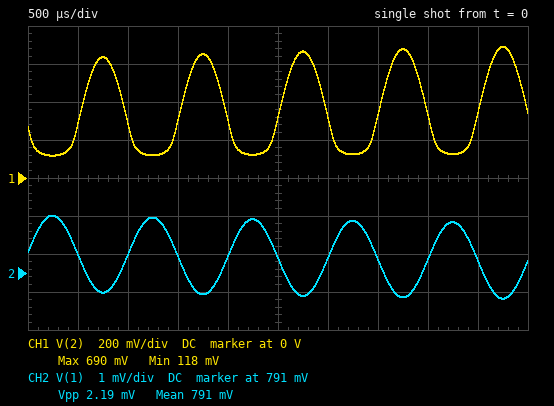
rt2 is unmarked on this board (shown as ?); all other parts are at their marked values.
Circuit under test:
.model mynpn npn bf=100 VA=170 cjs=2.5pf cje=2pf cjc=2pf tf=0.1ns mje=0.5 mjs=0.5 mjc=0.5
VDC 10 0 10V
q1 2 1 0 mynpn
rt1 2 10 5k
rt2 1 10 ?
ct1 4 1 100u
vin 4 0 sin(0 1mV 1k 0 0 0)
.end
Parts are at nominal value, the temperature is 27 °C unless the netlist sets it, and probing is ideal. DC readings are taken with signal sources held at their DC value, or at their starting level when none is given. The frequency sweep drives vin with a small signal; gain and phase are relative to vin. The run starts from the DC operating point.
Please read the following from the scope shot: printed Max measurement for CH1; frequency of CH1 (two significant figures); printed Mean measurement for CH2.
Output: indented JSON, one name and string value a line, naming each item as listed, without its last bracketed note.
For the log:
{
  "printed Max measurement for CH1": "690 mV",
  "frequency of CH1": "1.0 kHz",
  "printed Mean measurement for CH2": "791 mV"
}
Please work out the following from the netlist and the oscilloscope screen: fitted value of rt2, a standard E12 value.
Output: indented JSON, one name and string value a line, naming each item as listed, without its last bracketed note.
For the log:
{
  "fitted value of rt2, a standard E12 value": "470 kΩ"
}
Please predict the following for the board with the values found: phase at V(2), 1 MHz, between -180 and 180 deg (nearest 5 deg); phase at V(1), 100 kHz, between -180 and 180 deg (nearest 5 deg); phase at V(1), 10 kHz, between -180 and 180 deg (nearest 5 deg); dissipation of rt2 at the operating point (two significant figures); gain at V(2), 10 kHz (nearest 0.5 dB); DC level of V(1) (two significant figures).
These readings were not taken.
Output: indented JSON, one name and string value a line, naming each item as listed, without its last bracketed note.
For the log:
{
  "phase at V(2), 1 MHz, between -180 and 180 deg": "170 deg",
  "phase at V(1), 100 kHz, between -180 and 180 deg": "0 deg",
  "phase at V(1), 10 kHz, between -180 and 180 deg": "0 deg",
  "dissipation of rt2 at the operating point": "180 µW",
  "gain at V(2), 10 kHz": "51.0 dB",
  "DC level of V(1)": "790 mV"
}
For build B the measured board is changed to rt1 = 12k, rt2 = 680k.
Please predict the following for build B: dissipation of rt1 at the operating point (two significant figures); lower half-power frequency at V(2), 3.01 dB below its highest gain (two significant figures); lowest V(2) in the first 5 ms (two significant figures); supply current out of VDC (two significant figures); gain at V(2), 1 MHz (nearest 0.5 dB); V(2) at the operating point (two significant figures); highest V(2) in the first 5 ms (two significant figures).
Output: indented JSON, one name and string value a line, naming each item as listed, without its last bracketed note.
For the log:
{
  "dissipation of rt1 at the operating point": "8.1 mW",
  "lower half-power frequency at V(2), 3.01 dB below its highest gain": "22 Hz",
  "lowest V(2) in the first 5 ms": "98 mV",
  "supply current out of VDC": "840 µA",
  "gain at V(2), 1 MHz": "36.0 dB",
  "V(2) at the operating point": "130 mV",
  "highest V(2) in the first 5 ms": "410 mV"
}
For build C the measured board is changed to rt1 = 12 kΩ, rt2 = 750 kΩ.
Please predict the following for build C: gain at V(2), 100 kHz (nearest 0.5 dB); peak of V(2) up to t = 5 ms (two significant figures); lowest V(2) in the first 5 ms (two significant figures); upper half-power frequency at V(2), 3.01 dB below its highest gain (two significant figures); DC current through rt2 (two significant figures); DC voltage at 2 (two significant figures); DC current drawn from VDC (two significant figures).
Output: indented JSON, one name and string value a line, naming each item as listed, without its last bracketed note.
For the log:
{
  "gain at V(2), 100 kHz": "38.0 dB",
  "peak of V(2) up to t = 5 ms": "450 mV",
  "lowest V(2) in the first 5 ms": "100 mV",
  "upper half-power frequency at V(2), 3.01 dB below its highest gain": "10 MHz",
  "DC current through rt2": "12 µA",
  "DC voltage at 2": "140 mV",
  "DC current drawn from VDC": "830 µA"
}
